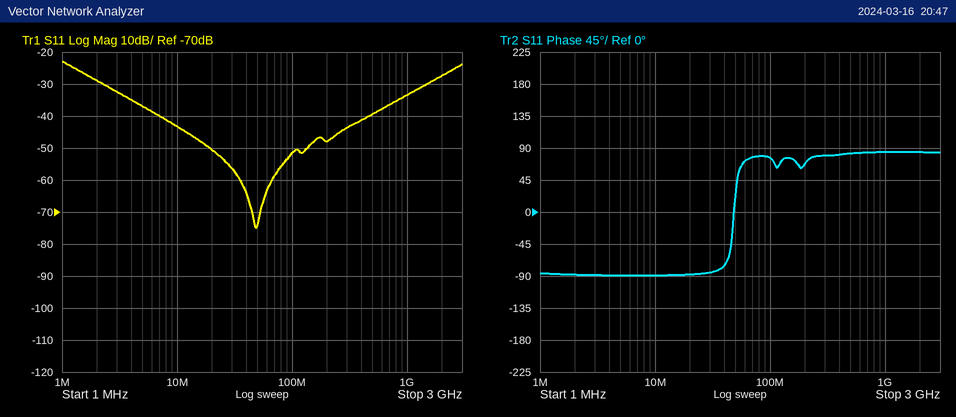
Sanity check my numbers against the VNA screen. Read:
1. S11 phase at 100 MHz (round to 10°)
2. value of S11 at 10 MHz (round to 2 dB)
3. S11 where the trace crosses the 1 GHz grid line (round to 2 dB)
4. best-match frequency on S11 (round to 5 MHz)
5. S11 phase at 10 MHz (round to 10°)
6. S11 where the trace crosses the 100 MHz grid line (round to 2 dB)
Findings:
80°
-44 dB
-34 dB
50 MHz
-90°
-52 dB
